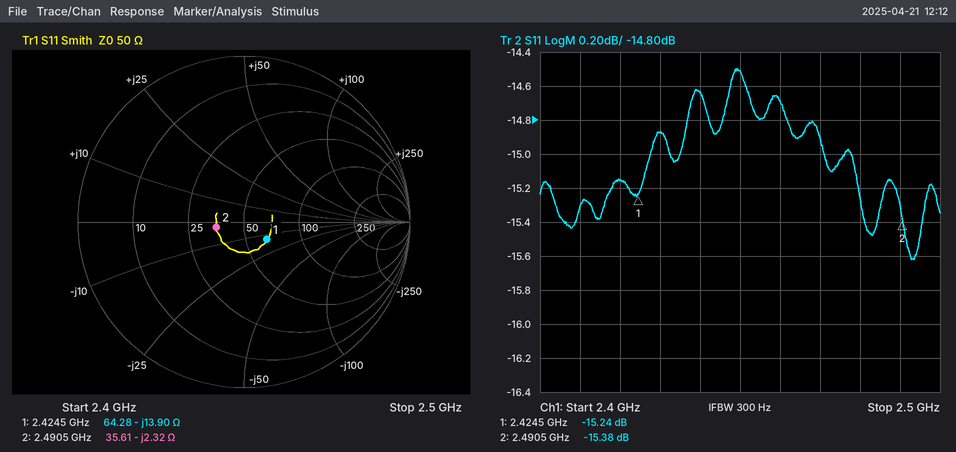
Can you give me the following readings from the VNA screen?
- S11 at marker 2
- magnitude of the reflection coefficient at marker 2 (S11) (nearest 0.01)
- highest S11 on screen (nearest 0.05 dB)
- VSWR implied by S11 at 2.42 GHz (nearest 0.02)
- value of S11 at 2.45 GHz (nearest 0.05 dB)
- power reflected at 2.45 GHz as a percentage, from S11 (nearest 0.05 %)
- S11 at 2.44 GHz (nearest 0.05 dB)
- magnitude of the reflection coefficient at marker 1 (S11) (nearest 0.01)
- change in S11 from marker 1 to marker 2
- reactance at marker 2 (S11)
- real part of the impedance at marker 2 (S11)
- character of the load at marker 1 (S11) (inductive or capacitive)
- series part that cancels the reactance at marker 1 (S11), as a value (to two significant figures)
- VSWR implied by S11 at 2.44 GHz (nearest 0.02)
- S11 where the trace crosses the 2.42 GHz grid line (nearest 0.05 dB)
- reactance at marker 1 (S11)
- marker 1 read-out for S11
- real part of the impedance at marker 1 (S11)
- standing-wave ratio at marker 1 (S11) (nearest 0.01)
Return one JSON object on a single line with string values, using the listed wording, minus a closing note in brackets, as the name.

{"S11 at marker 2": "-15.38 dB", "magnitude of the reflection coefficient at marker 2 (S11)": "0.17", "highest S11 on screen": "-14.50 dB", "VSWR implied by S11 at 2.42 GHz": "1.42", "value of S11 at 2.45 GHz": "-14.50 dB", "power reflected at 2.45 GHz as a percentage, from S11": "3.55 %", "S11 at 2.44 GHz": "-14.65 dB", "magnitude of the reflection coefficient at marker 1 (S11)": "0.17", "change in S11 from marker 1 to marker 2": "-0.14 dB", "reactance at marker 2": "-2.32 Ω", "real part of the impedance at marker 2": "35.61 Ω", "character of the load at marker 1 (S11)": "capacitive", "series part that cancels the reactance at marker 1 (S11), as a value": "910 pH", "VSWR implied by S11 at 2.44 GHz": "1.46", "S11 where the trace crosses the 2.42 GHz grid line": "-15.15 dB", "reactance at marker 1": "-13.90 Ω", "marker 1 read-out for S11": "-15.24 dB", "real part of the impedance at marker 1": "64.28 Ω", "standing-wave ratio at marker 1 (S11)": "1.42"}
